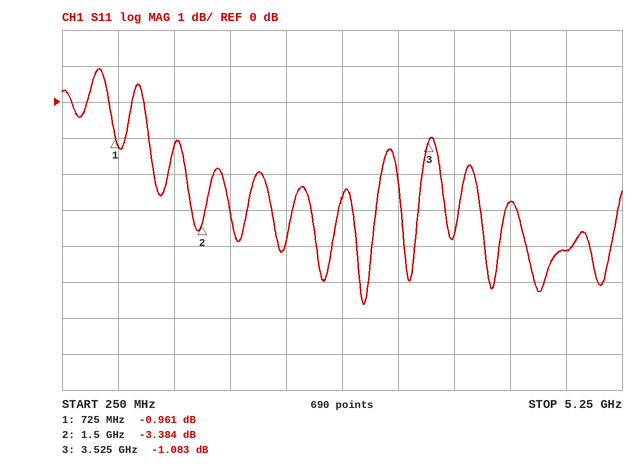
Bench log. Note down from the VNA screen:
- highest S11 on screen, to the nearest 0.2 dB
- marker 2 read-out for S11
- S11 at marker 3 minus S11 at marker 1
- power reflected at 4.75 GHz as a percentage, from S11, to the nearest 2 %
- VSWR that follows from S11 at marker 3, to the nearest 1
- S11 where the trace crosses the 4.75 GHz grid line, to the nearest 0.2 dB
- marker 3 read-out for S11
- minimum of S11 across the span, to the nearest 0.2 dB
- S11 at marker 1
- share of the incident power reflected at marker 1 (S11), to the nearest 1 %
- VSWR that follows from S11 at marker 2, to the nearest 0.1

1.0 dB
-3.384 dB
-0.122 dB
38 %
16
-4.2 dB
-1.083 dB
-5.6 dB
-0.961 dB
80 %
5.2
